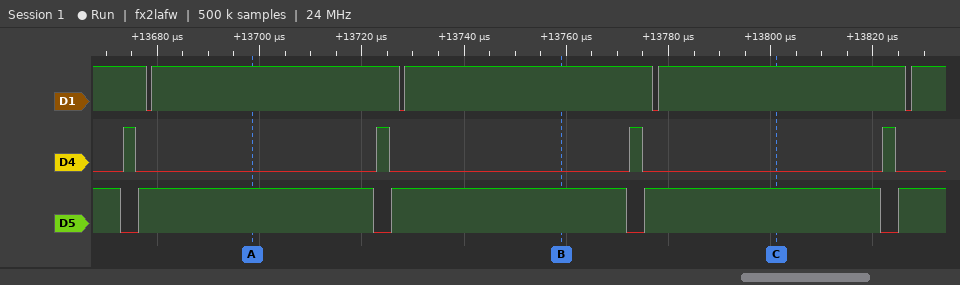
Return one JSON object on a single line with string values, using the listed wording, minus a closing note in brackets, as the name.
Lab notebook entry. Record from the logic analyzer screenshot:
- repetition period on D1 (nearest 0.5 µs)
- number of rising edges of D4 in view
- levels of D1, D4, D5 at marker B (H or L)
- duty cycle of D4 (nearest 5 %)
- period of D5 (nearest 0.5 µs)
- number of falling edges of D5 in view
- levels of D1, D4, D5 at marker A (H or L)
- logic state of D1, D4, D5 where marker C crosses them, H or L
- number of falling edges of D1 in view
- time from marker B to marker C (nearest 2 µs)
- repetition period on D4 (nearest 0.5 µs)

{"repetition period on D1": "49.5 µs", "number of rising edges of D4 in view": "4", "levels of D1, D4, D5 at marker B": "D1=H, D4=L, D5=H", "duty cycle of D4": "5 %", "period of D5": "49.5 µs", "number of falling edges of D5 in view": "4", "levels of D1, D4, D5 at marker A": "D1=H, D4=L, D5=H", "logic state of D1, D4, D5 where marker C crosses them, H or L": "D1=H, D4=L, D5=H", "number of falling edges of D1 in view": "4", "time from marker B to marker C": "42 µs", "repetition period on D4": "49.5 µs"}
